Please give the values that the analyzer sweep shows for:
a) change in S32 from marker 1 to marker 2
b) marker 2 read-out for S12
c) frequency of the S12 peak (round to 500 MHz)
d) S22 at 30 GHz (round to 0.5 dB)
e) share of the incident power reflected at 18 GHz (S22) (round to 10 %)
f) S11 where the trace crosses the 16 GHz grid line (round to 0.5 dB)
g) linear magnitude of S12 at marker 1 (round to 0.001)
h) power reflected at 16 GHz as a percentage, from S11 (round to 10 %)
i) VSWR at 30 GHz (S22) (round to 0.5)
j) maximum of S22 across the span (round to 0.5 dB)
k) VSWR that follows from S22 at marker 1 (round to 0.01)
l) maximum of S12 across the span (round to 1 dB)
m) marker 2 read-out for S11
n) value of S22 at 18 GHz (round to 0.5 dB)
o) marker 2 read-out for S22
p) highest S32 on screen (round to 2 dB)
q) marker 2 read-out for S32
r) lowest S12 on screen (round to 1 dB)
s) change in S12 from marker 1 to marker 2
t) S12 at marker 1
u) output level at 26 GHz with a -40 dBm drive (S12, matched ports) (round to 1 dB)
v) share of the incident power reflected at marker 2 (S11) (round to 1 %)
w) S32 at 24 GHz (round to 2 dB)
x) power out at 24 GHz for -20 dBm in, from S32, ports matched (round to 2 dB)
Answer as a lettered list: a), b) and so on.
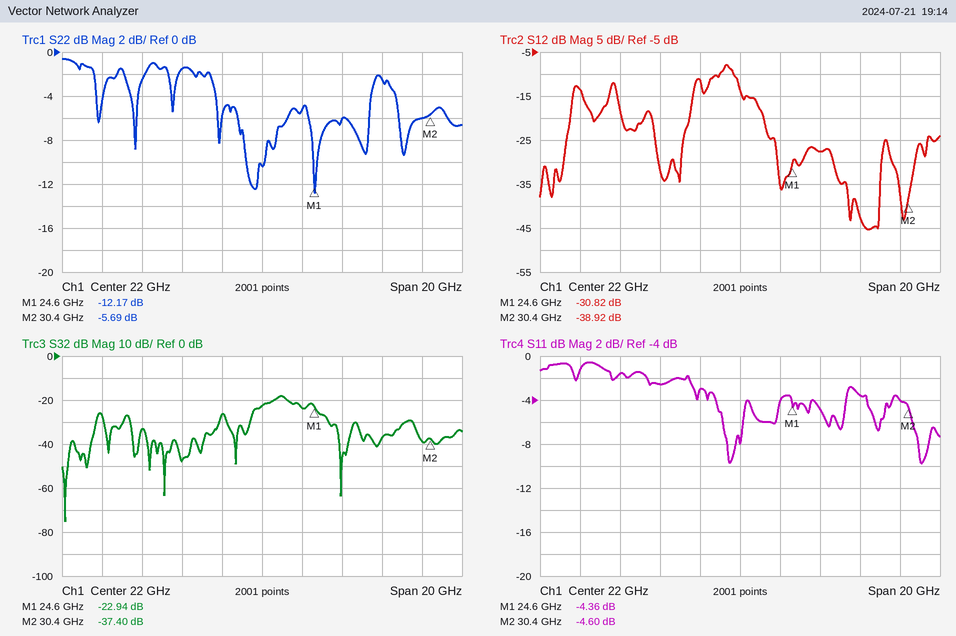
a) -14.46 dB
b) -38.92 dB
c) 21.5 GHz
d) -6.0 dB
e) 70 %
f) -1.5 dB
g) 0.029
h) 70 %
i) 3.0
j) -0.5 dB
k) 1.65
l) -8 dB
m) -4.60 dB
n) -1.5 dB
o) -5.69 dB
p) -18 dB
q) -37.40 dB
r) -45 dB
s) -8.10 dB
t) -30.82 dB
u) -68 dBm
v) 35 %
w) -24 dB
x) -44 dBm
